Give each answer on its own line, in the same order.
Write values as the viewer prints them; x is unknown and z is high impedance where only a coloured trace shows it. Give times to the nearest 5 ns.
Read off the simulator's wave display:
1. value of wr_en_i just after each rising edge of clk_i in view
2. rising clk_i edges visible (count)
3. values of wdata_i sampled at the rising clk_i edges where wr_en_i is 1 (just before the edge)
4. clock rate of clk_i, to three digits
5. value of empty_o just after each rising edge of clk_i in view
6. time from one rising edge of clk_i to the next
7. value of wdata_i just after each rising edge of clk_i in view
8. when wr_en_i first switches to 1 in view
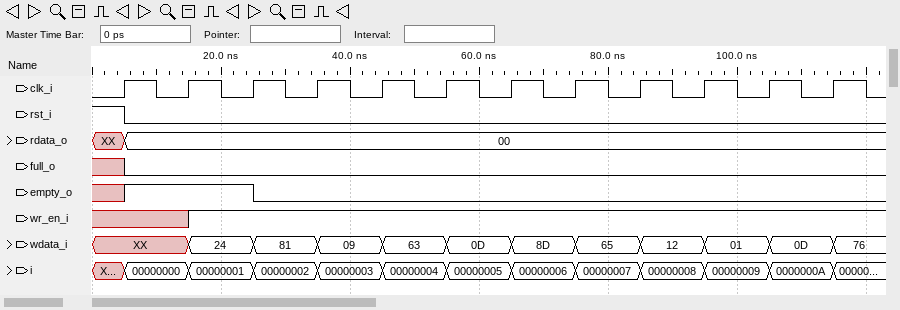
x 1 1 1 1 1 1 1 1 1 1 1
12
24, 81, 09, 63, 0D, 8D, 65, 12, 01, 0D
100 MHz
1 1 0 0 0 0 0 0 0 0 0 0
10 ns
XX, 24, 81, 09, 63, 0D, 8D, 65, 12, 01, 0D, 76
15 ns
